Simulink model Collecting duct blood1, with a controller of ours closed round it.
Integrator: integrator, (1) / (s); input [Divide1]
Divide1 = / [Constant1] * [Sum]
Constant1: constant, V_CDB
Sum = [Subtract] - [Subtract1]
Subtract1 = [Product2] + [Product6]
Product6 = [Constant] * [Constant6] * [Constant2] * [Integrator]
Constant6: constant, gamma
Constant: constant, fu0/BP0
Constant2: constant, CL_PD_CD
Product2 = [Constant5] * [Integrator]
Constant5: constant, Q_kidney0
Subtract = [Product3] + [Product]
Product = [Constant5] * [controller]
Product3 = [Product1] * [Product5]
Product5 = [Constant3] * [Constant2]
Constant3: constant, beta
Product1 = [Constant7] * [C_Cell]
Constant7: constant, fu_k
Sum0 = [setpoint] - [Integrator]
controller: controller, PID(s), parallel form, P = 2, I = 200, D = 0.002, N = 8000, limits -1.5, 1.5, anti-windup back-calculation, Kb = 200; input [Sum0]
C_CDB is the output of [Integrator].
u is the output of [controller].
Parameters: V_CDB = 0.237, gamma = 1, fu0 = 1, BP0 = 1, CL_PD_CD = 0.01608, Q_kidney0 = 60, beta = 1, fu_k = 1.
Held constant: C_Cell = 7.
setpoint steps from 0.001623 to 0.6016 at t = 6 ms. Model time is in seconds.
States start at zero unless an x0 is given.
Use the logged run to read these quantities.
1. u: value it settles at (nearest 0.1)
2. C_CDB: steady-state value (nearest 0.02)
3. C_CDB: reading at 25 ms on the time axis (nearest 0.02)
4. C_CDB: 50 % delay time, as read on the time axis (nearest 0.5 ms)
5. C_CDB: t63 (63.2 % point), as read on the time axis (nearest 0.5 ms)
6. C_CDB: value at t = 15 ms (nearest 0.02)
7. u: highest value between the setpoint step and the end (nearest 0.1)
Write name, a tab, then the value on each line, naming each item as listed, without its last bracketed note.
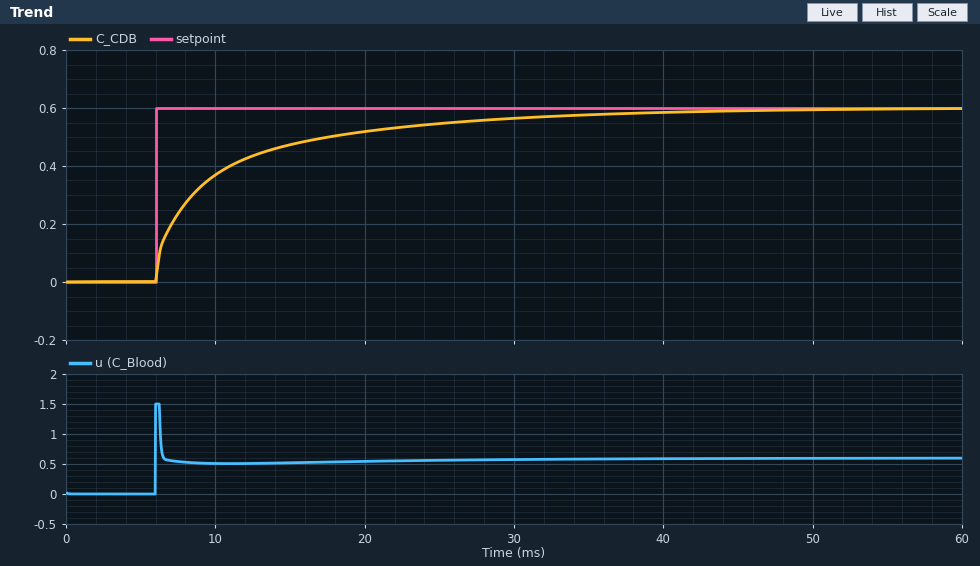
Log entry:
u: value it settles at	0.6
C_CDB: steady-state value	0.60
C_CDB: reading at 25 ms on the time axis	0.54
C_CDB: 50 % delay time, as read on the time axis	8.5 ms
C_CDB: t63 (63.2 % point), as read on the time axis	10.5 ms
C_CDB: value at t = 15 ms	0.48
u: highest value between the setpoint step and the end	1.5
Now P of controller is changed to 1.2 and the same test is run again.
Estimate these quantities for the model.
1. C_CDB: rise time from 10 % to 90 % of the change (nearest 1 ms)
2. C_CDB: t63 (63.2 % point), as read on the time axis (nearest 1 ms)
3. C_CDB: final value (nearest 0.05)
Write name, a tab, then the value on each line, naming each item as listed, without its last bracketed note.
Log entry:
C_CDB: rise time from 10 % to 90 % of the change	15 ms
C_CDB: t63 (63.2 % point), as read on the time axis	12 ms
C_CDB: final value	0.60
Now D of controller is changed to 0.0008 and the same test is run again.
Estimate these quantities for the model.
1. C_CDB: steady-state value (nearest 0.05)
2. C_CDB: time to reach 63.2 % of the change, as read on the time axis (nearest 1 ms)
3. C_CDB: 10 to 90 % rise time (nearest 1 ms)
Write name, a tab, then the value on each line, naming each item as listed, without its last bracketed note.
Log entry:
C_CDB: steady-state value	0.60
C_CDB: time to reach 63.2 % of the change, as read on the time axis	9 ms
C_CDB: 10 to 90 % rise time	16 ms
